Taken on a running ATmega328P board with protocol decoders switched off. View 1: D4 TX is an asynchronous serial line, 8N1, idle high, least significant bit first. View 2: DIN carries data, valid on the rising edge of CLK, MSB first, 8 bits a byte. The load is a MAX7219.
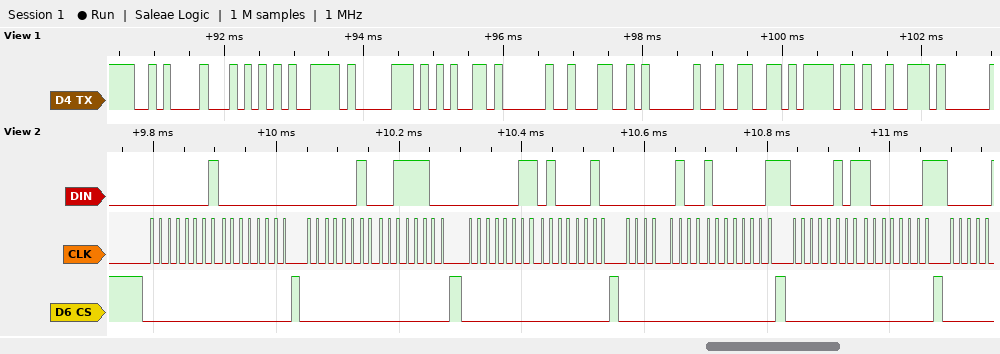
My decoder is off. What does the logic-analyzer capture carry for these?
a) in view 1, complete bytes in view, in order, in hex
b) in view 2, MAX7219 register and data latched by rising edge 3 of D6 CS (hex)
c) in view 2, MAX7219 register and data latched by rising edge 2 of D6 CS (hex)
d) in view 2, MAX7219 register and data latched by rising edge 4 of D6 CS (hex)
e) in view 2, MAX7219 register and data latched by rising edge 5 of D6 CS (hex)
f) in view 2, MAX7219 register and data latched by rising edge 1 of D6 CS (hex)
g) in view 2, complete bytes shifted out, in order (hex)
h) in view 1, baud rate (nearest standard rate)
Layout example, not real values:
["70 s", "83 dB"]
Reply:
["0A 54 79 70 65 20 4C 20 66 6F 72", "register 0x3, data 0x42", "register 0x2, data 0x3C", "register 0x4, data 0x81", "register 0x5, data 0x81", "register 0x1, data 0x00", "0x01 0x00 0x02 0x3C 0x03 0x42 0x04 0x81 0x05 0x81", "9600 baud"]
